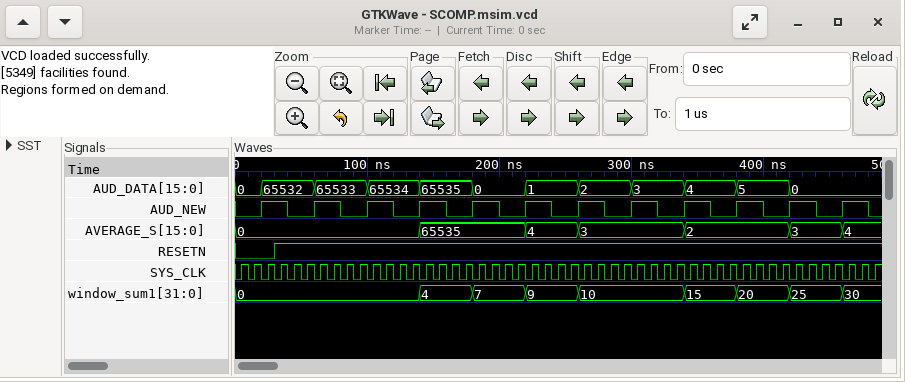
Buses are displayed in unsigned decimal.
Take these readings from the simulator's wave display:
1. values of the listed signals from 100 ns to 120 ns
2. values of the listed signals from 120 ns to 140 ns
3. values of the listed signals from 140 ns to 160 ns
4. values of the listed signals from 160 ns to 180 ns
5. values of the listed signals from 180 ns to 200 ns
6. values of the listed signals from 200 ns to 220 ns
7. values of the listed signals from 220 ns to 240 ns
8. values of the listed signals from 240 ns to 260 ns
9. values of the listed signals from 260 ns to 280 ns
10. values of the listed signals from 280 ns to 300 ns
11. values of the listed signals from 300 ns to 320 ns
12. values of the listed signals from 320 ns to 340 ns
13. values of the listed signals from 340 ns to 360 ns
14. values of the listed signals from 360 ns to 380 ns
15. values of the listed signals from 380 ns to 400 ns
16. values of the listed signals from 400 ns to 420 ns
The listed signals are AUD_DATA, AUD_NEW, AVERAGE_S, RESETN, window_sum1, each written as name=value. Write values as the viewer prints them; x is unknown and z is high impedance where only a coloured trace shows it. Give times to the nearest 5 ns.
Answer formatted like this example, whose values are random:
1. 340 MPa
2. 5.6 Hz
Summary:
1. AUD_DATA=65534, AUD_NEW=1, AVERAGE_S=0, RESETN=1, window_sum1=0
2. AUD_DATA=65534, AUD_NEW=0, AVERAGE_S=0, RESETN=1, window_sum1=0
3. AUD_DATA=65535, AUD_NEW=1, AVERAGE_S=65535, RESETN=1, window_sum1=4
4. AUD_DATA=65535, AUD_NEW=0, AVERAGE_S=65535, RESETN=1, window_sum1=4
5. AUD_DATA=0, AUD_NEW=1, AVERAGE_S=65535, RESETN=1, window_sum1=7
6. AUD_DATA=0, AUD_NEW=0, AVERAGE_S=65535, RESETN=1, window_sum1=7
7. AUD_DATA=1, AUD_NEW=1, AVERAGE_S=4, RESETN=1, window_sum1=9
8. AUD_DATA=1, AUD_NEW=0, AVERAGE_S=4, RESETN=1, window_sum1=9
9. AUD_DATA=2, AUD_NEW=1, AVERAGE_S=3, RESETN=1, window_sum1=10
10. AUD_DATA=2, AUD_NEW=0, AVERAGE_S=3, RESETN=1, window_sum1=10
11. AUD_DATA=3, AUD_NEW=1, AVERAGE_S=3, RESETN=1, window_sum1=10
12. AUD_DATA=3, AUD_NEW=0, AVERAGE_S=3, RESETN=1, window_sum1=10
13. AUD_DATA=4, AUD_NEW=1, AVERAGE_S=2, RESETN=1, window_sum1=15
14. AUD_DATA=4, AUD_NEW=0, AVERAGE_S=2, RESETN=1, window_sum1=15
15. AUD_DATA=5, AUD_NEW=1, AVERAGE_S=2, RESETN=1, window_sum1=20
16. AUD_DATA=5, AUD_NEW=0, AVERAGE_S=2, RESETN=1, window_sum1=20
